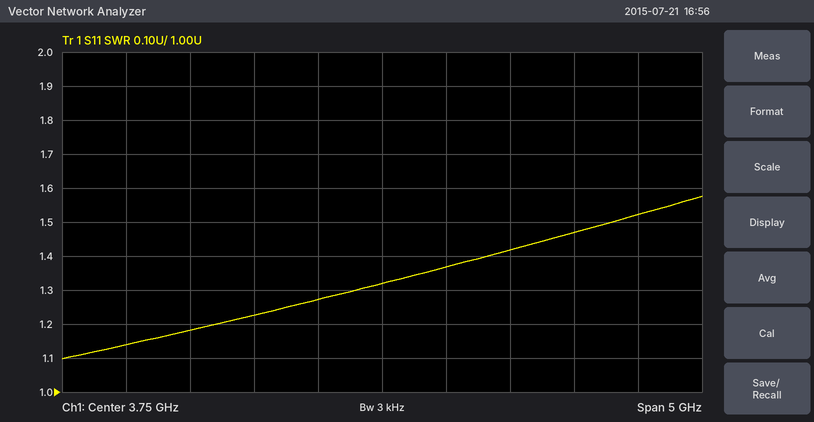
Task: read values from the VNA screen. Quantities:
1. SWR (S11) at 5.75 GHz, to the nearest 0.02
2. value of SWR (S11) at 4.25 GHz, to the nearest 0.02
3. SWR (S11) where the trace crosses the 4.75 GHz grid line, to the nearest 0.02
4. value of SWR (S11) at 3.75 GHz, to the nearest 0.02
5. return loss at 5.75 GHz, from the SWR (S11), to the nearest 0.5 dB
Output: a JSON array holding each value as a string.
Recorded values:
["1.52", "1.36", "1.42", "1.32", "13.5 dB"]
